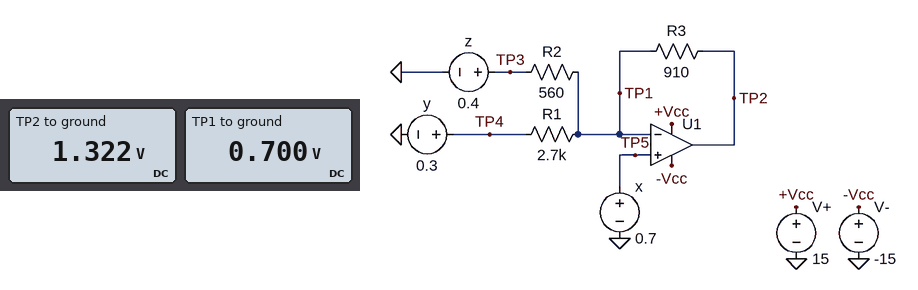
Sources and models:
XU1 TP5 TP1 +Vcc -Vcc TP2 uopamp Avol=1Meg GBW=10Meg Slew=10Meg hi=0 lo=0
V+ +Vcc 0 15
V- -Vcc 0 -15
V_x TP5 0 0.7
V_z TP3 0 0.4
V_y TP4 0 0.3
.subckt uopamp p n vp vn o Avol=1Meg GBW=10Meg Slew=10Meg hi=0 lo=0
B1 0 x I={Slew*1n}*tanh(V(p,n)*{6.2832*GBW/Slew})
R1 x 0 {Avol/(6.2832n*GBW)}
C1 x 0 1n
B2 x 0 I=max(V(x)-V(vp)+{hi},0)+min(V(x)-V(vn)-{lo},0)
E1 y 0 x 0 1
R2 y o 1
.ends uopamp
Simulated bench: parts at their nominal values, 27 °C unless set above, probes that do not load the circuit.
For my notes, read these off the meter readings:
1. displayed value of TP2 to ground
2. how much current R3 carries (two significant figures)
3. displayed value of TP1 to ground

1.322 V
680 µA
0.700 V
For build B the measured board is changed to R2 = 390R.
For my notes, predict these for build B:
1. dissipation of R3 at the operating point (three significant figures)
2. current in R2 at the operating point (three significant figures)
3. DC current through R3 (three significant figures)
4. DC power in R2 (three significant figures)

766 µW
769 µA
917 µA
231 µW
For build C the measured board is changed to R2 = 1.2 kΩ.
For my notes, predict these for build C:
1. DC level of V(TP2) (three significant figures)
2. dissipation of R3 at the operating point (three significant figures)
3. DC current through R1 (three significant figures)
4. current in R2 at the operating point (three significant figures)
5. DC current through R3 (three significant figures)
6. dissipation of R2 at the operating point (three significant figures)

1.06 V
144 µW
148 µA
250 µA
398 µA
75.0 µW
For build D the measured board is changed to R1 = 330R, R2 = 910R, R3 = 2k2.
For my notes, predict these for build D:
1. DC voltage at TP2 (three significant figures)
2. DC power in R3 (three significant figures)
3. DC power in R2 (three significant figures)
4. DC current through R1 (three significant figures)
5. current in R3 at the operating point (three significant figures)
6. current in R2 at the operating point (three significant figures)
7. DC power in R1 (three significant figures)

4.09 V
5.23 mW
98.9 µW
1.21 mA
1.54 mA
330 µA
485 µW
